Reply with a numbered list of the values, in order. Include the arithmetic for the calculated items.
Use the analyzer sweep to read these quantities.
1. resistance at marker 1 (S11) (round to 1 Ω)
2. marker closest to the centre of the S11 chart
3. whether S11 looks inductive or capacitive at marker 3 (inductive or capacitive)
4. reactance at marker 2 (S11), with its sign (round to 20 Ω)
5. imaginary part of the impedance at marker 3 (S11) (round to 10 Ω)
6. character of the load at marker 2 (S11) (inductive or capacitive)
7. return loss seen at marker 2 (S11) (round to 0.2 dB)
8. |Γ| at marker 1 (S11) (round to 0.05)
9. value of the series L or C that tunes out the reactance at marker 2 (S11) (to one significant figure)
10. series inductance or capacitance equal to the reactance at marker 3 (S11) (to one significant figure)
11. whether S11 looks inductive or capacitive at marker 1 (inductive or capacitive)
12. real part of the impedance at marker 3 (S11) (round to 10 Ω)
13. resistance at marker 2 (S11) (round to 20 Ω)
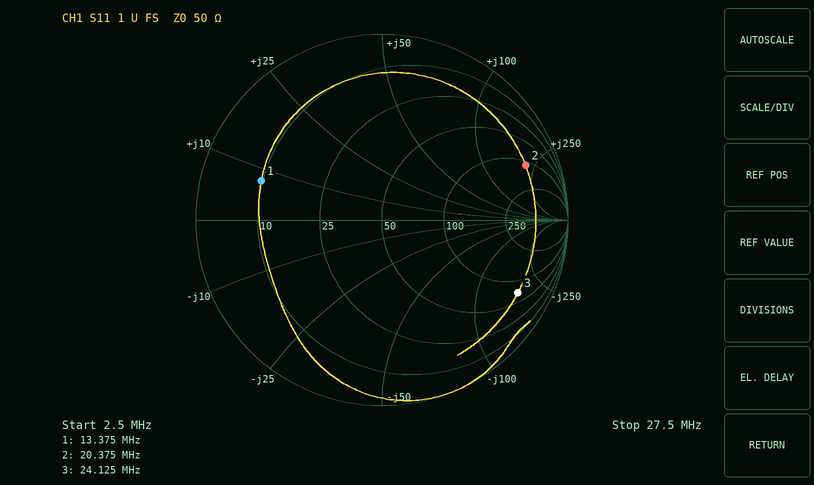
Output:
1. 10 Ω
2. marker 1
3. capacitive
4. +220 Ω
5. -170 Ω
6. inductive
7. 1.6 dB
8. 0.70
9. C = 1/(2π × 20.375 MHz × 220 Ω) ≈ 35.5 pF, so 40 pF to one significant figure
10. C = 1/(2π × 24.125 MHz × 170 Ω) ≈ 38.8 pF, so 40 pF to one significant figure
11. inductive
12. 70 Ω
13. 120 Ω
